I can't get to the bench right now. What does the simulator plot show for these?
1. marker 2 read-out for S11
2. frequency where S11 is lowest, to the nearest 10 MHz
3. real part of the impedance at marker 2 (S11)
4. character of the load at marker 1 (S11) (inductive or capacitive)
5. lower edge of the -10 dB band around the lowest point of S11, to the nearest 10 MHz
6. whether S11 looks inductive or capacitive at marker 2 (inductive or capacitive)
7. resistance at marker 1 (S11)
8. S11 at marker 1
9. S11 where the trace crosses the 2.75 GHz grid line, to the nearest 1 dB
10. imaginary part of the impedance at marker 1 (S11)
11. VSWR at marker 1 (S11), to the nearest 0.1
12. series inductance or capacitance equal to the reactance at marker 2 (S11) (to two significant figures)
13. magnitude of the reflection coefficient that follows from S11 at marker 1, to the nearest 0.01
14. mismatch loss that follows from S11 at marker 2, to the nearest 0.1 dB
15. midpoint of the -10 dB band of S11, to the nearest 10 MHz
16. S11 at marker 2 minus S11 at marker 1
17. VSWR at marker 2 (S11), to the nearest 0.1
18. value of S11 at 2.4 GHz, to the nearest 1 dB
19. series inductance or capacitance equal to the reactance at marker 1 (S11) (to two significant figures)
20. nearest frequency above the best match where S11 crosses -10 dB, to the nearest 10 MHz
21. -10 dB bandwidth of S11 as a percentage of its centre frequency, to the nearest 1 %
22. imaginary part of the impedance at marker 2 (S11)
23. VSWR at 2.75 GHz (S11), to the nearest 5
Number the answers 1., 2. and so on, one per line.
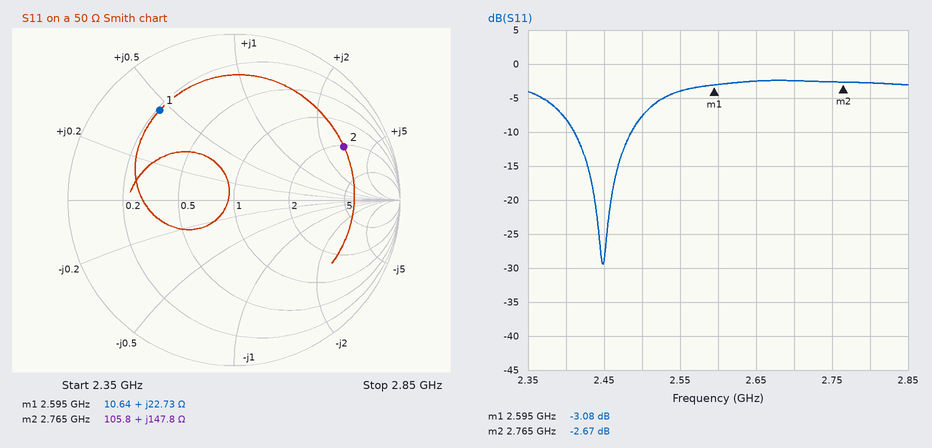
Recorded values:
1. -2.67 dB
2. 2.45 GHz
3. 105.8 Ω
4. inductive
5. 2.41 GHz
6. inductive
7. 10.64 Ω
8. -3.08 dB
9. -3 dB
10. +22.73 Ω
11. 5.7
12. 8.5 nH
13. 0.70
14. 3.4 dB
15. 2.45 GHz
16. 0.41 dB
17. 6.6
18. -8 dB
19. 1.4 nH
20. 2.49 GHz
21. 3 %
22. +147.8 Ω
23. 5
